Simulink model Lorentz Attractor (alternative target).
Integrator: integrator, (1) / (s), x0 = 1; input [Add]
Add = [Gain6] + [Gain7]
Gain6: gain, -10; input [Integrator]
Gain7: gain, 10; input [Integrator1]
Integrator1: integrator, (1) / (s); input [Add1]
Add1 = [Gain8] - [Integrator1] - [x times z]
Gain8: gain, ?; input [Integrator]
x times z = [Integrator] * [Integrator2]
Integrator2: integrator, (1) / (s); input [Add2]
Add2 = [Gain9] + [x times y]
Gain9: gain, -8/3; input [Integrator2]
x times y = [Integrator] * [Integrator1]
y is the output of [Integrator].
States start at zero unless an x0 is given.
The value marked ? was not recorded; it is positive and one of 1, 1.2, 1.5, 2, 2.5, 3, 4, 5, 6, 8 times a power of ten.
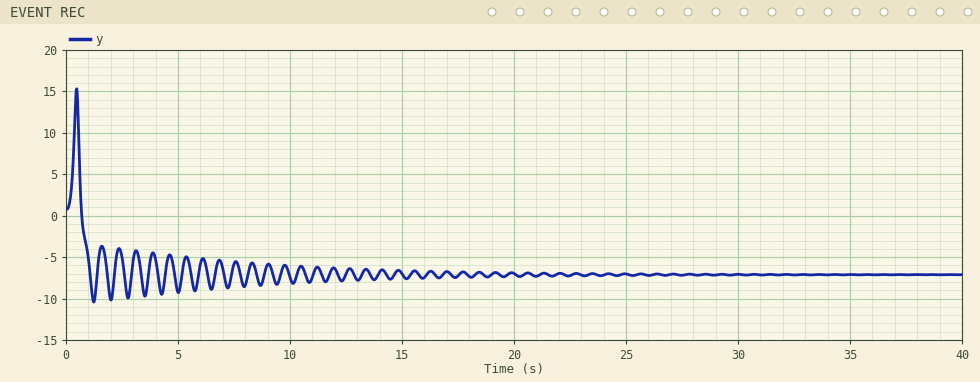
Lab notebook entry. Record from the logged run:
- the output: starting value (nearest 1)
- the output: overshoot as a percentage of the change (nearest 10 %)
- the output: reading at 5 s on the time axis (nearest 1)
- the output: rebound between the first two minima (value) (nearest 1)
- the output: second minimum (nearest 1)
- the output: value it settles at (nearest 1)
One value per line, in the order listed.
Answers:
1
40 %
-9
-4
-10
-7
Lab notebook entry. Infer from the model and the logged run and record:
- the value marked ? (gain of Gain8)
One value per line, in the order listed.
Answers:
20
